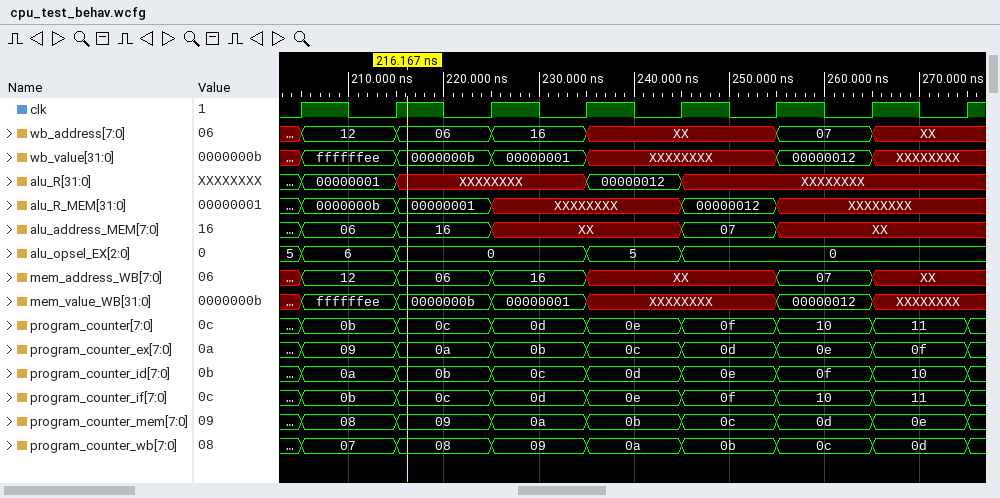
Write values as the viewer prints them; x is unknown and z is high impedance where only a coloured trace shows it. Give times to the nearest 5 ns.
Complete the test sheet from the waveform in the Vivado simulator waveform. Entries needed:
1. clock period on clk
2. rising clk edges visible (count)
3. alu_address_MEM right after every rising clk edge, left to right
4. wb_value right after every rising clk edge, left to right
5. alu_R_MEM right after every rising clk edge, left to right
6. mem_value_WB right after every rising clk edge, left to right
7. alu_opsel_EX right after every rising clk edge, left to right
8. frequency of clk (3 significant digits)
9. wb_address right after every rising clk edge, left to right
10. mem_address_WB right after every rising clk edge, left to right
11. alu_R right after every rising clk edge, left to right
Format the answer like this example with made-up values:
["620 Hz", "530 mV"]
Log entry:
["10 ns", "8", "06, 16, XX, XX, 07, XX, XX, XX", "ffffffee, 0000000b, 00000001, XXXXXXXX, XXXXXXXX, 00000012, XXXXXXXX, XXXXXXXX", "0000000b, 00000001, XXXXXXXX, XXXXXXXX, 00000012, XXXXXXXX, XXXXXXXX, XXXXXXXX", "ffffffee, 0000000b, 00000001, XXXXXXXX, XXXXXXXX, 00000012, XXXXXXXX, XXXXXXXX", "6, 0, 0, 5, 0, 0, 0, 0", "100 MHz", "12, 06, 16, XX, XX, 07, XX, XX", "12, 06, 16, XX, XX, 07, XX, XX", "00000001, XXXXXXXX, XXXXXXXX, 00000012, XXXXXXXX, XXXXXXXX, XXXXXXXX, XXXXXXXX"]
